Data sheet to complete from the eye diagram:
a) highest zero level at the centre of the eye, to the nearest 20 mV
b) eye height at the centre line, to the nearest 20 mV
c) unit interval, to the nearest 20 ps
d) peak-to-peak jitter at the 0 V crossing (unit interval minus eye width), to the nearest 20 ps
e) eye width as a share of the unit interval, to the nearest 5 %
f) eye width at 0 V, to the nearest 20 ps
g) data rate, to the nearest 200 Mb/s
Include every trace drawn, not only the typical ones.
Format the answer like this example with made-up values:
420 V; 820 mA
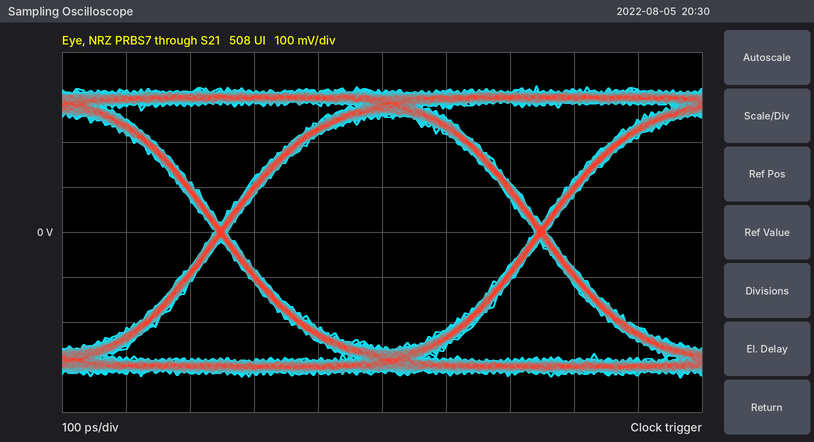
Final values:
-260 mV; 520 mV; 500 ps; 20 ps; 95 %; 480 ps; 2.0 Gb/s
